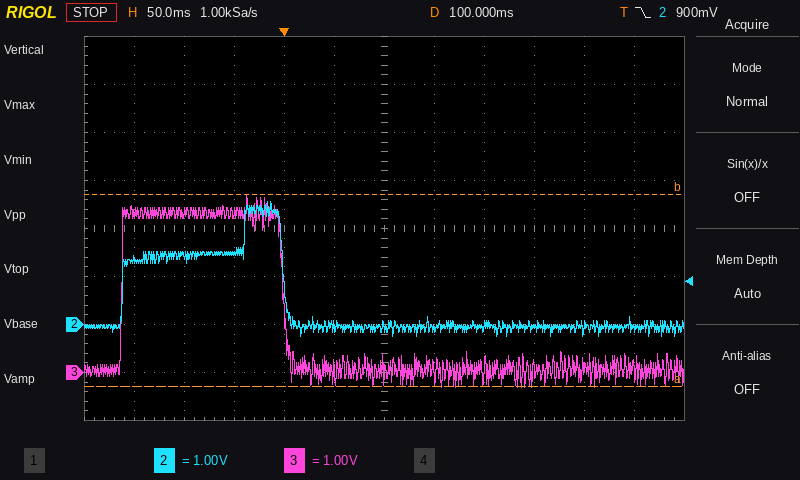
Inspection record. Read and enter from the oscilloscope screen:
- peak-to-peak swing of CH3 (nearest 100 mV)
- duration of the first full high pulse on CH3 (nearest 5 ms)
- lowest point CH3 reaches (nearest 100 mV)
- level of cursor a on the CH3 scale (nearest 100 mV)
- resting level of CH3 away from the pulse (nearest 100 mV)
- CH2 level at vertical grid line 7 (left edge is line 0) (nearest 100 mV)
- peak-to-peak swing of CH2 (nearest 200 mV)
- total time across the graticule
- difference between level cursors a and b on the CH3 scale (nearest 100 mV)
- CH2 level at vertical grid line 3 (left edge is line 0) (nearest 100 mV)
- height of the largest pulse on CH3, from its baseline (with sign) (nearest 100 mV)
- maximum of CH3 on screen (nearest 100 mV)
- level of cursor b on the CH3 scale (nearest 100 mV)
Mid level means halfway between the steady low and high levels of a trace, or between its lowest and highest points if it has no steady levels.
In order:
4.0 V
160 ms
-300 mV
-300 mV
100 mV
-100 mV
2.8 V
600 ms
4.0 V
1.5 V
+3.6 V
3.7 V
3.7 V
